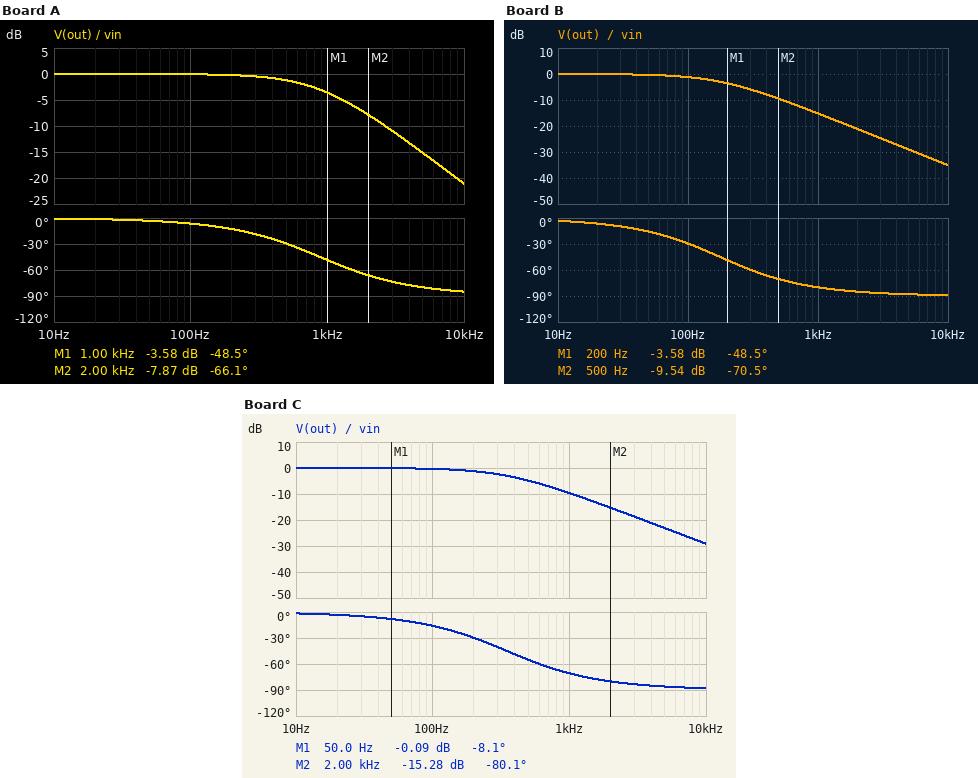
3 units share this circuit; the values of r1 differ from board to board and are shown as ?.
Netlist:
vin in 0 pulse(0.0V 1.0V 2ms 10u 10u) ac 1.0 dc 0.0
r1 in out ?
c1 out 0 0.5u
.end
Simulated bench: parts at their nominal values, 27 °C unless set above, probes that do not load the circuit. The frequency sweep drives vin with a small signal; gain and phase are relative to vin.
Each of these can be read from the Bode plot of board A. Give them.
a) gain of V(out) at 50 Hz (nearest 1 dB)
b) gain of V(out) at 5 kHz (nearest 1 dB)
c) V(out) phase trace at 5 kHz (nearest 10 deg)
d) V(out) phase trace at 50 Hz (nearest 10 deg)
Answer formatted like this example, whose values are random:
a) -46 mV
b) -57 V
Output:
a) 0 dB
b) -15 dB
c) -80 deg
d) 0 deg
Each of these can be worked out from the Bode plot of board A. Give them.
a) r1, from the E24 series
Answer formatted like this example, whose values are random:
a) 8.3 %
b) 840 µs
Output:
a) 360 Ω
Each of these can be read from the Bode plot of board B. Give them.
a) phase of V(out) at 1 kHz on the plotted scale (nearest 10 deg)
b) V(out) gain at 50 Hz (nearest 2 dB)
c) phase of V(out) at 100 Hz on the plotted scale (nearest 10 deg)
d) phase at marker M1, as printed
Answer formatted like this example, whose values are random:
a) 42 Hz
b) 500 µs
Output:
a) -80 deg
b) 0 dB
c) -30 deg
d) -48.5 deg
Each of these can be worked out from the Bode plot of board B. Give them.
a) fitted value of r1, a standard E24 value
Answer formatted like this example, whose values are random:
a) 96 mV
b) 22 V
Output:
a) 1.8 kΩ
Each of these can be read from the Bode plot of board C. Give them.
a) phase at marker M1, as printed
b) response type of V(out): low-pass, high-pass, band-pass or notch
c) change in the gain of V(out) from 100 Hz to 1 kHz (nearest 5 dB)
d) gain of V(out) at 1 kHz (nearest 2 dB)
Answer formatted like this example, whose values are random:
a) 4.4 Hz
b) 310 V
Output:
a) -8.1 deg
b) low-pass
c) -10 dB
d) -10 dB
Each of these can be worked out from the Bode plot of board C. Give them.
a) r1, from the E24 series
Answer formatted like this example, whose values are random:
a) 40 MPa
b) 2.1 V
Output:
a) 910 Ω
